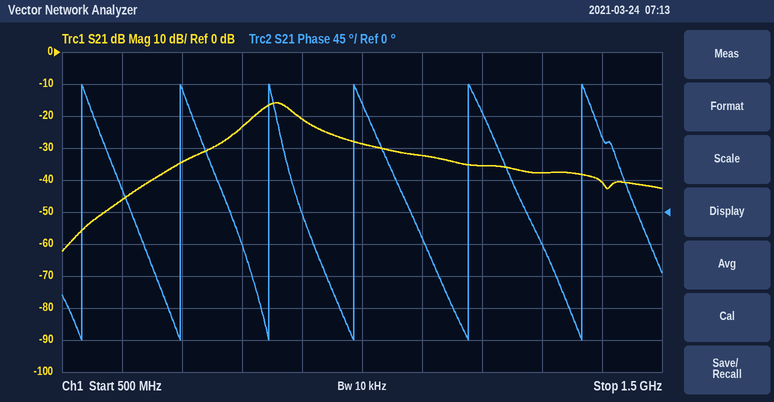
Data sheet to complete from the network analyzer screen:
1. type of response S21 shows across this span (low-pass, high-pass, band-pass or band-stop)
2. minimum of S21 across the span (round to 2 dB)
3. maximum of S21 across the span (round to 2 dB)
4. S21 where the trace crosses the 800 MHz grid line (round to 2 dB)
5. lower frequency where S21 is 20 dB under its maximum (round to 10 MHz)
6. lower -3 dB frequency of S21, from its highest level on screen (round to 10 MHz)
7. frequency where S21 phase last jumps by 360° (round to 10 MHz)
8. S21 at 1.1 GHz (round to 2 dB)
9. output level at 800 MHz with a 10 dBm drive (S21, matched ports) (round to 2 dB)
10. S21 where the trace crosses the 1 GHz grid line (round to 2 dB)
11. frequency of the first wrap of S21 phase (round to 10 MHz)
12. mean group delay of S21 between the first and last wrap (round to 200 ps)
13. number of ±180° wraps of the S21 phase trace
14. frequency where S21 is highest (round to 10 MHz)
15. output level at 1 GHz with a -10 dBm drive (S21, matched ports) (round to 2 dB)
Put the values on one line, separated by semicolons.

band-pass; -62 dB; -16 dB; -24 dB; 690 MHz; 830 MHz; 1.37 GHz; -32 dB; -14 dBm; -28 dB; 530 MHz; 6.0 ns; 6; 860 MHz; -38 dBm
